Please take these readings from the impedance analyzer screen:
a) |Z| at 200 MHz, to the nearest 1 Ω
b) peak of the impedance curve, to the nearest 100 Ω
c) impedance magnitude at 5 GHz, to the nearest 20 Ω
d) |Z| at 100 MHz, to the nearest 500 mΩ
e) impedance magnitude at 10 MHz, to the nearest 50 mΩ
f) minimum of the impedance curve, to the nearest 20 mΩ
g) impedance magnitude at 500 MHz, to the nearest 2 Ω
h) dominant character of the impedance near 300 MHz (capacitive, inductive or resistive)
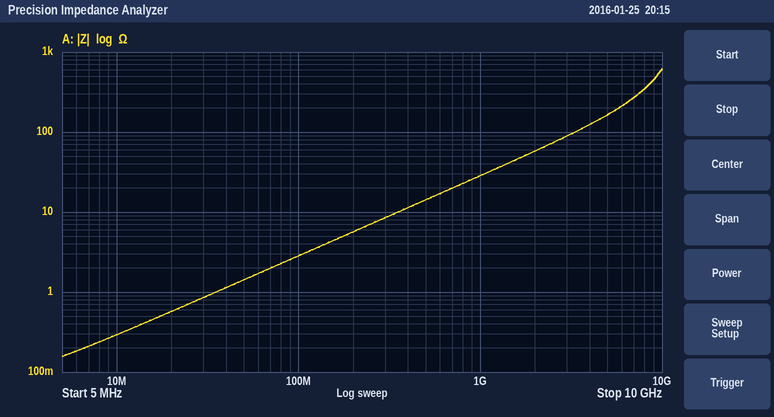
6 Ω
600 Ω
160 Ω
3.0 Ω
300 mΩ
160 mΩ
14 Ω
inductive
